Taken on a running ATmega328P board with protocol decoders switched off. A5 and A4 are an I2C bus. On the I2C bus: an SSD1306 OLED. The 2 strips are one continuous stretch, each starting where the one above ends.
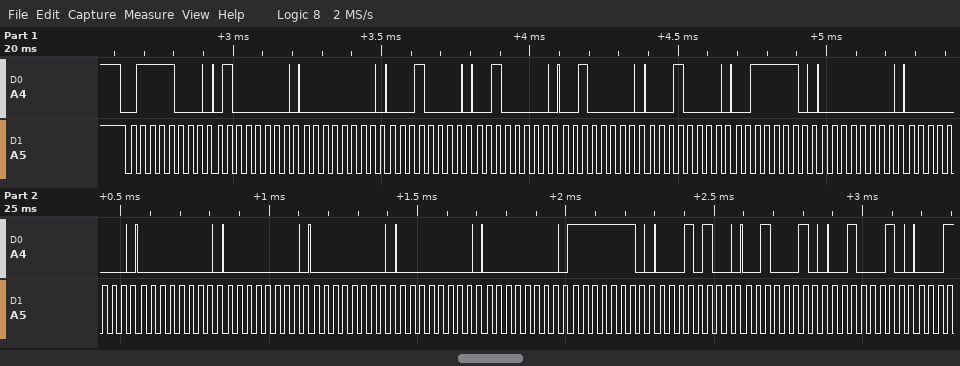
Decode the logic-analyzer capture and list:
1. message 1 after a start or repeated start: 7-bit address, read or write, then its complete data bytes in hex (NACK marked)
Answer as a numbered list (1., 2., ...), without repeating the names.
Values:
1. 0x3C write: 40 00 10 20 20 10 3E 00 00 00 00 00 00 00 FE 14 22 22
